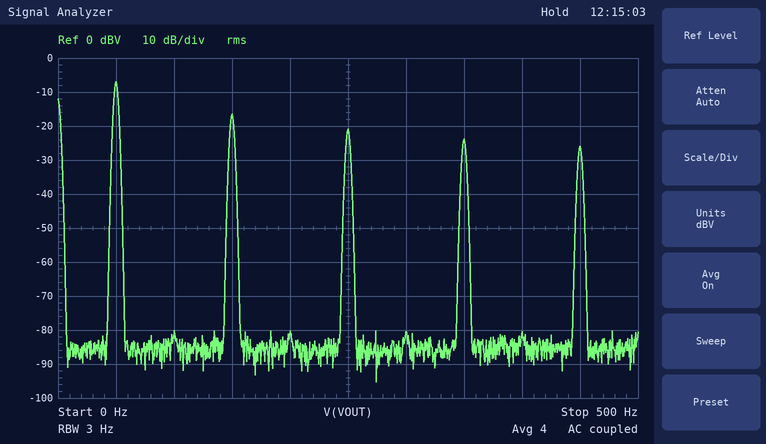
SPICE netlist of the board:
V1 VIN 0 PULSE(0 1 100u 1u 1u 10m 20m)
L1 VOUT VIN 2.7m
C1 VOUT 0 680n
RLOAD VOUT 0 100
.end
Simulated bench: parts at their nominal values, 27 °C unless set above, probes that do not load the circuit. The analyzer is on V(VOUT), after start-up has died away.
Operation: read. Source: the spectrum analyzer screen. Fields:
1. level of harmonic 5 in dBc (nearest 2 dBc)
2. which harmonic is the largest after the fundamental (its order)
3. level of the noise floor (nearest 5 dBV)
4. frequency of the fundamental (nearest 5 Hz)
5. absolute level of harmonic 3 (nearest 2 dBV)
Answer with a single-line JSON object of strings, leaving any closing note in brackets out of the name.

{"level of harmonic 5 in dBc": "-14 dBc", "which harmonic is the largest after the fundamental": "3", "level of the noise floor": "-85 dBV", "frequency of the fundamental": "50 Hz", "absolute level of harmonic 3": "-16 dBV"}
